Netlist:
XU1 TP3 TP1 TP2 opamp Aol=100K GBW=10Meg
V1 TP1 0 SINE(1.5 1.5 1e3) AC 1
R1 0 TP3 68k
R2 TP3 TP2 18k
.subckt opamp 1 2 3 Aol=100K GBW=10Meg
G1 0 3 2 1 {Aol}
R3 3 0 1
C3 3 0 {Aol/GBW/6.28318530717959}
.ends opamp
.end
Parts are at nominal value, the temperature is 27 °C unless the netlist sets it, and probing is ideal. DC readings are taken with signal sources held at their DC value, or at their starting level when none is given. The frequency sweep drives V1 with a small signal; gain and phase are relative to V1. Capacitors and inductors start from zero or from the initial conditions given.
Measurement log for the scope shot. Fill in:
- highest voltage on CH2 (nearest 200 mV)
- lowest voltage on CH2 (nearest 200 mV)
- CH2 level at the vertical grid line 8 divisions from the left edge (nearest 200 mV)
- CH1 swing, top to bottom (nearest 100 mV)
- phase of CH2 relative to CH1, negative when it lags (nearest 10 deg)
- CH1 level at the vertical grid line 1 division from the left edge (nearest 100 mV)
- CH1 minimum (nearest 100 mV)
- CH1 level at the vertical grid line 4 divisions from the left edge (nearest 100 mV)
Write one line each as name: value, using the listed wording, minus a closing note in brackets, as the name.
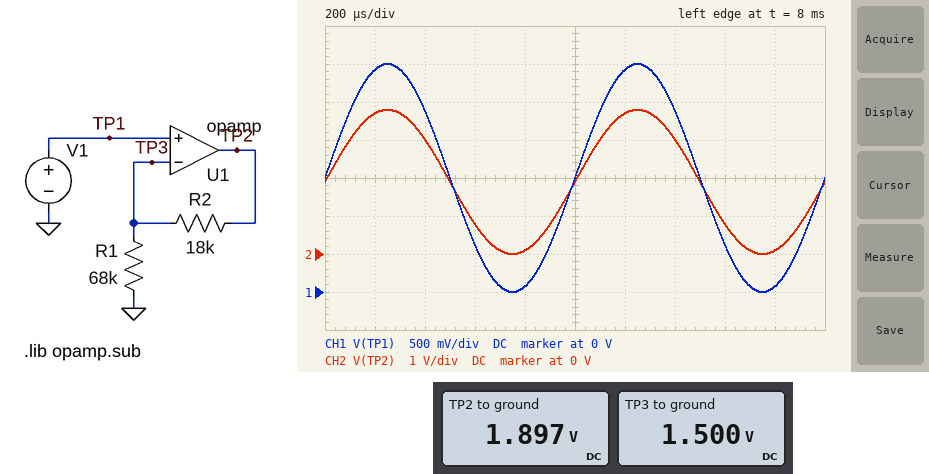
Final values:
highest voltage on CH2: 3.8 V
lowest voltage on CH2: 0 V
CH2 level at the vertical grid line 8 divisions from the left edge: 800 mV
CH1 swing, top to bottom: 3.0 V
phase of CH2 relative to CH1, negative when it lags: 0 deg
CH1 level at the vertical grid line 1 division from the left edge: 2.9 V
CH1 minimum: 0 V
CH1 level at the vertical grid line 4 divisions from the left edge: 100 mV
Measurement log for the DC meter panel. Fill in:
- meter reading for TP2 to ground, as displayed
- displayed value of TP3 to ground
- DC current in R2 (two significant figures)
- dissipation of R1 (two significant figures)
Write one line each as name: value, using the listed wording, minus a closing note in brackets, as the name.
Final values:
meter reading for TP2 to ground, as displayed: 1.897 V
displayed value of TP3 to ground: 1.500 V
DC current in R2: 22 µA
dissipation of R1: 33 µW
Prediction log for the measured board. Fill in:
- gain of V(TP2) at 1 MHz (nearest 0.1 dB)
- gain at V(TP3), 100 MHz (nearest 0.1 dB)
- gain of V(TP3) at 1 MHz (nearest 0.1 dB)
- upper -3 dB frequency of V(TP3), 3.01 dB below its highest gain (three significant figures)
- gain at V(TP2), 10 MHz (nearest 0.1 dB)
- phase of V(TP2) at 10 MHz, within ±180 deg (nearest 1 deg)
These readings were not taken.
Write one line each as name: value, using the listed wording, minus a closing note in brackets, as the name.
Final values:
gain of V(TP2) at 1 MHz: 2.0 dB
gain at V(TP3), 100 MHz: -22.1 dB
gain of V(TP3) at 1 MHz: -0.1 dB
upper -3 dB frequency of V(TP3), 3.01 dB below its highest gain: 7.91 MHz
gain at V(TP2), 10 MHz: -2.1 dB
phase of V(TP2) at 10 MHz, within ±180 deg: -52 deg
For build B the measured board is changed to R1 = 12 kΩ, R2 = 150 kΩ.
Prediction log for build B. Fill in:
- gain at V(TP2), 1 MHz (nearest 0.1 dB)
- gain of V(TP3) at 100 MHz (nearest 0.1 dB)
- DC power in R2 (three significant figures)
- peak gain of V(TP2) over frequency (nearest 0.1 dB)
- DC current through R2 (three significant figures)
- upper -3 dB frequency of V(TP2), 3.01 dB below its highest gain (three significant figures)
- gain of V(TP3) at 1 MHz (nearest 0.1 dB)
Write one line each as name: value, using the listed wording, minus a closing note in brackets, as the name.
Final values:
gain at V(TP2), 1 MHz: 18.1 dB
gain of V(TP3) at 100 MHz: -42.6 dB
DC power in R2: 2.34 mW
peak gain of V(TP2) over frequency: 22.6 dB
DC current through R2: 125 µA
upper -3 dB frequency of V(TP2), 3.01 dB below its highest gain: 741 kHz
gain of V(TP3) at 1 MHz: -4.5 dB
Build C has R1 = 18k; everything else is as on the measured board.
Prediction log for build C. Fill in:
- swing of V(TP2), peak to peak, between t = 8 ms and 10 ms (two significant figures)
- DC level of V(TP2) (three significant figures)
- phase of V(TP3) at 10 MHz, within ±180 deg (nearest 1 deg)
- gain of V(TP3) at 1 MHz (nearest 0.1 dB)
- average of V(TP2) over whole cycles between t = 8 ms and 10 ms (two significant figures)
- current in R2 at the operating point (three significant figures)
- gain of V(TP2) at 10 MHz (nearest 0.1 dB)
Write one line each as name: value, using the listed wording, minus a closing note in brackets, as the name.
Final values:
swing of V(TP2), peak to peak, between t = 8 ms and 10 ms: 6.0 V
DC level of V(TP2): 3.00 V
phase of V(TP3) at 10 MHz, within ±180 deg: -63 deg
gain of V(TP3) at 1 MHz: -0.2 dB
average of V(TP2) over whole cycles between t = 8 ms and 10 ms: 3.0 V
current in R2 at the operating point: 83.3 µA
gain of V(TP2) at 10 MHz: -1.0 dB
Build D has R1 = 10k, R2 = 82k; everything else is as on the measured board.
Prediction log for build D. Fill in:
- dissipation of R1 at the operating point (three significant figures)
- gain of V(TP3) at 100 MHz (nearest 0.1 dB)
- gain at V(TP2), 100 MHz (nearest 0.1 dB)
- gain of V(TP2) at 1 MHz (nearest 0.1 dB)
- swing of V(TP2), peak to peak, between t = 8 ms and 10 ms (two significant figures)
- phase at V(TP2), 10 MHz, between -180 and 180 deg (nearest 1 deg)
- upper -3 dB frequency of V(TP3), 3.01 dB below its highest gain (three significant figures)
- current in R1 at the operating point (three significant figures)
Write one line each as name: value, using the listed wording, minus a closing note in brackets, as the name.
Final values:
dissipation of R1 at the operating point: 225 µW
gain of V(TP3) at 100 MHz: -39.3 dB
gain at V(TP2), 100 MHz: -20.0 dB
gain of V(TP2) at 1 MHz: 16.6 dB
swing of V(TP2), peak to peak, between t = 8 ms and 10 ms: 28 V
phase at V(TP2), 10 MHz, between -180 and 180 deg: -84 deg
upper -3 dB frequency of V(TP3), 3.01 dB below its highest gain: 1.09 MHz
current in R1 at the operating point: 150 µA
